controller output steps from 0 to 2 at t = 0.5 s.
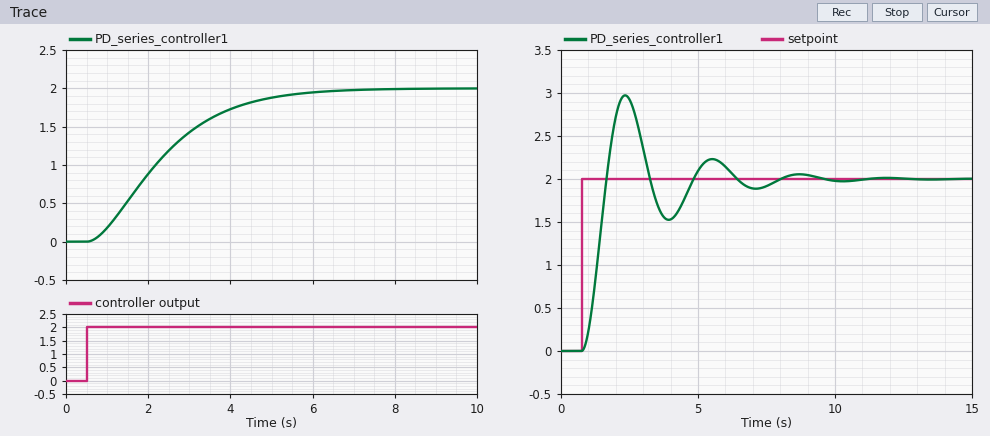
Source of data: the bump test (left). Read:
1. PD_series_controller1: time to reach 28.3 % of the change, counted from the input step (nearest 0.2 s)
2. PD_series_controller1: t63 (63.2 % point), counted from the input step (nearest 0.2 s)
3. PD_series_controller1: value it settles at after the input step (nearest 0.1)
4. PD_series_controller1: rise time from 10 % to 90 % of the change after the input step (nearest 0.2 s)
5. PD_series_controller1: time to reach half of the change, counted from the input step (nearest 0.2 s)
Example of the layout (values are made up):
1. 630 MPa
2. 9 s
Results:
1. 1.0 s
2. 2.2 s
3. 2.0
4. 3.4 s
5. 1.6 s
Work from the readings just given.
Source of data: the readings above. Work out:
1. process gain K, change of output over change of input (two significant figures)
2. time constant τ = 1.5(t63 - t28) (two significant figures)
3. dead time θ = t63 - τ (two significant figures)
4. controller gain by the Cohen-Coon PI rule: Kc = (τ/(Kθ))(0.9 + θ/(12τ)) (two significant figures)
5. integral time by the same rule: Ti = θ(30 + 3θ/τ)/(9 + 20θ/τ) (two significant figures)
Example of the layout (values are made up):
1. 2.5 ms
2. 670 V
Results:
1. 1.0
2. 1.8 s
3. 0.40 s
4. 4.1
5. 0.91 s
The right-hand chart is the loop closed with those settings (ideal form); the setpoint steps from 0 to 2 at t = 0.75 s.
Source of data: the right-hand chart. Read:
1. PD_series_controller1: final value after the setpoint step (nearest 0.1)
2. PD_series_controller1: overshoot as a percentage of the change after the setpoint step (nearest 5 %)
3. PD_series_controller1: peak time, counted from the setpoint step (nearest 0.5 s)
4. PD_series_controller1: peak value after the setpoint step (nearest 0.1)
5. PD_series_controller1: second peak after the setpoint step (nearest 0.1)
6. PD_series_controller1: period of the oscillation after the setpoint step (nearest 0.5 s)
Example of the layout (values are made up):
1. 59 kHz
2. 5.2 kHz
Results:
1. 2.0
2. 50 %
3. 1.5 s
4. 3.0
5. 2.2
6. 3.0 s
